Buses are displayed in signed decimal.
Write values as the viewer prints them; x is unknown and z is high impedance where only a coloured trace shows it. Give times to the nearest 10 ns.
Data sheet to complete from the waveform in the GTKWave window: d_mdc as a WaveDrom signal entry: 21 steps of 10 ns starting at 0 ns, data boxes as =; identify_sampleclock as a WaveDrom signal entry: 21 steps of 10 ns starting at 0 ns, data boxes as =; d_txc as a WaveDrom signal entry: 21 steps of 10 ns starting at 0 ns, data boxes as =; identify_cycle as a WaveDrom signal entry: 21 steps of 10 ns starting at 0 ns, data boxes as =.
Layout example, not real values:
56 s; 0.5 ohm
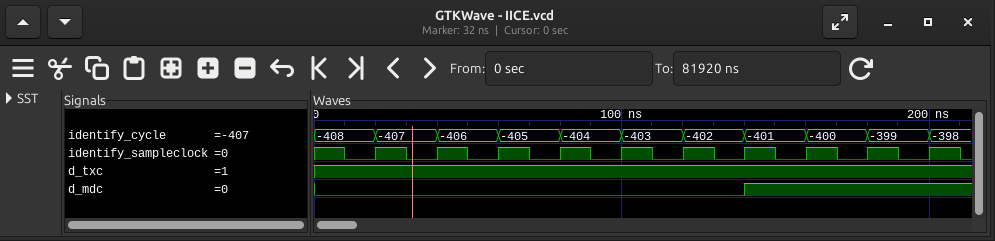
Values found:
{name: 'd_mdc', wave: '0.............1......'}; {name: 'identify_sampleclock', wave: '101010101010101010101'}; {name: 'd_txc', wave: '1....................'}; {name: 'identify_cycle', wave: '=.=.=.=.=.=.=.=.=.=.=', data: '-408 -407 -406 -405 -404 -403 -402 -401 -400 -399 -398'}
